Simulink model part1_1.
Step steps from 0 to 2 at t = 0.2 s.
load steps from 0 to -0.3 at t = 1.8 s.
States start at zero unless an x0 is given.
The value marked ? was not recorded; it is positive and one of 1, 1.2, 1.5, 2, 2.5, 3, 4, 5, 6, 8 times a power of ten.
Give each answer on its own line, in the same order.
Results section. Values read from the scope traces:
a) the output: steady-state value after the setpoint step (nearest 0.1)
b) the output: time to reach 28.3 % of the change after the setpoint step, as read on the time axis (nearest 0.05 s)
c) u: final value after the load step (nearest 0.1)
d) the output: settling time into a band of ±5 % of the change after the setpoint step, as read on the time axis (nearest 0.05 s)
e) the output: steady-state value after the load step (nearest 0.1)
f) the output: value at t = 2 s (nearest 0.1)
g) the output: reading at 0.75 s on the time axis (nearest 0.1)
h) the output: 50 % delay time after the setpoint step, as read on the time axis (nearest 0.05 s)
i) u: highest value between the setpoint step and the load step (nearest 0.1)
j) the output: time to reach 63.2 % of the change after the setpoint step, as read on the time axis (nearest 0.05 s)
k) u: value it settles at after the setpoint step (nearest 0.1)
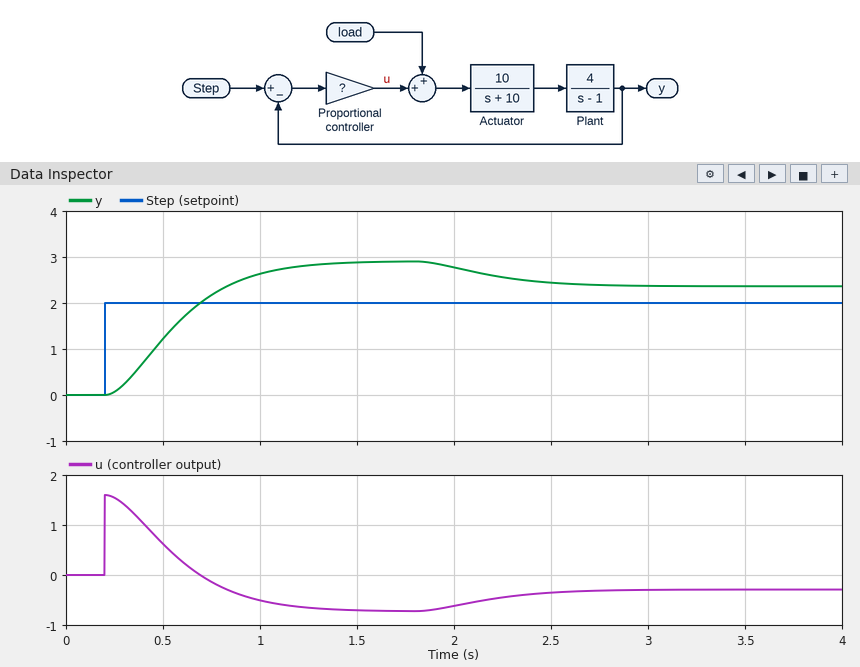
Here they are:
2.9
0.40 s
-0.3
1.15 s
2.4
2.8
2.2
0.55 s
1.6
0.65 s
-0.7
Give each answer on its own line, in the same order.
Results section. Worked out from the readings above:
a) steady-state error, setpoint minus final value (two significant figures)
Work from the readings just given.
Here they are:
-0.90
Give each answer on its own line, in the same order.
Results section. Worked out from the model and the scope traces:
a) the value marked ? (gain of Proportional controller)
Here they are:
0.8
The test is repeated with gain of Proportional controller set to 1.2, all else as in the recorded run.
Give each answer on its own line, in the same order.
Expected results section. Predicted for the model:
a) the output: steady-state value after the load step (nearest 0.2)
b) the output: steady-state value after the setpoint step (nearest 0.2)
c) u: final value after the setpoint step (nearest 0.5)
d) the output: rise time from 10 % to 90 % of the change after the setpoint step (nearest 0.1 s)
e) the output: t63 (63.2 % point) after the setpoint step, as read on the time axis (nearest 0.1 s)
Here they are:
2.2
2.6
-0.5
0.4 s
0.5 s
